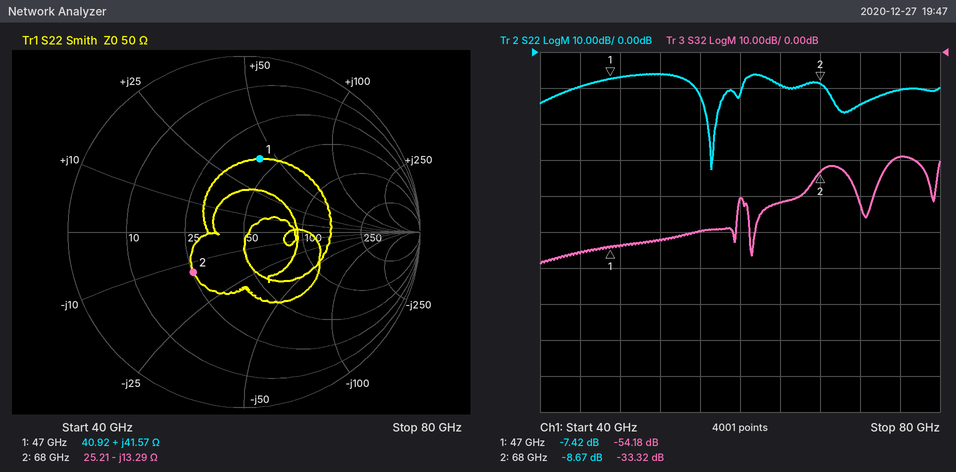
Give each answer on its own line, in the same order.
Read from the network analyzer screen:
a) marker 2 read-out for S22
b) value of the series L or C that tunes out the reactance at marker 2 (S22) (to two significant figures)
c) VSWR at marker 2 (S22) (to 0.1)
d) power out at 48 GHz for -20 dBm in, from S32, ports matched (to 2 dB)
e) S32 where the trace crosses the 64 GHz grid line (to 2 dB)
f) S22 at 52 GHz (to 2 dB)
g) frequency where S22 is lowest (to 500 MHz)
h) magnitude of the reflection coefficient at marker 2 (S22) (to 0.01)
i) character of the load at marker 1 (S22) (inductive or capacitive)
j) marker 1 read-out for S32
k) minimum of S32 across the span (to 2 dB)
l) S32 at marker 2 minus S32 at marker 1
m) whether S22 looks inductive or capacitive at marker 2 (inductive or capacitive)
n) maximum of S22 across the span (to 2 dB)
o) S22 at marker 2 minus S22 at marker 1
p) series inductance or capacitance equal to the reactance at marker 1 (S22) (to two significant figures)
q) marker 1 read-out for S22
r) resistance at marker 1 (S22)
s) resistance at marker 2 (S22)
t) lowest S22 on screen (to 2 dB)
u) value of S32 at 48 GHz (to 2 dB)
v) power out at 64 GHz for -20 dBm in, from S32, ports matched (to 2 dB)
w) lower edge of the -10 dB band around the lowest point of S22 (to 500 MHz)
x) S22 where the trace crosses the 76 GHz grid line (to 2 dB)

-8.67 dB
31 pH
2.2
-74 dBm
-42 dB
-6 dB
57.0 GHz
0.37
inductive
-54.18 dB
-58 dB
20.86 dB
capacitive
-6 dB
-1.25 dB
140 pH
-7.42 dB
40.92 Ω
25.21 Ω
-32 dB
-54 dB
-62 dBm
55.5 GHz
-10 dB
